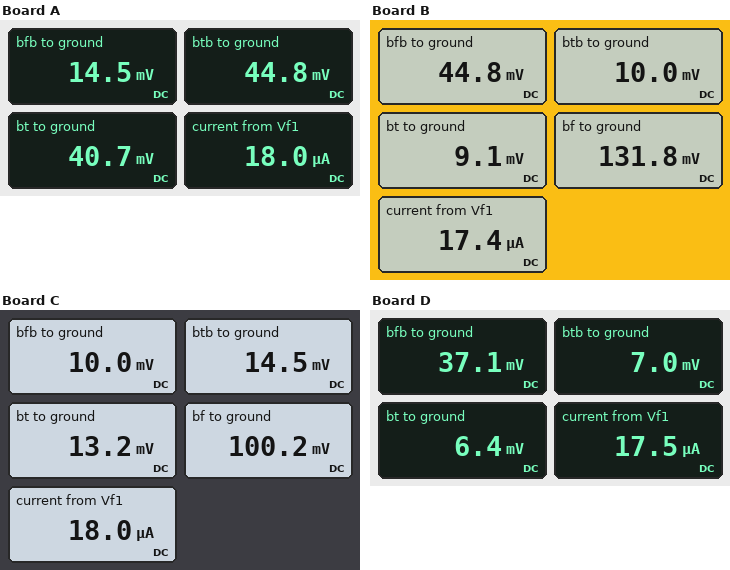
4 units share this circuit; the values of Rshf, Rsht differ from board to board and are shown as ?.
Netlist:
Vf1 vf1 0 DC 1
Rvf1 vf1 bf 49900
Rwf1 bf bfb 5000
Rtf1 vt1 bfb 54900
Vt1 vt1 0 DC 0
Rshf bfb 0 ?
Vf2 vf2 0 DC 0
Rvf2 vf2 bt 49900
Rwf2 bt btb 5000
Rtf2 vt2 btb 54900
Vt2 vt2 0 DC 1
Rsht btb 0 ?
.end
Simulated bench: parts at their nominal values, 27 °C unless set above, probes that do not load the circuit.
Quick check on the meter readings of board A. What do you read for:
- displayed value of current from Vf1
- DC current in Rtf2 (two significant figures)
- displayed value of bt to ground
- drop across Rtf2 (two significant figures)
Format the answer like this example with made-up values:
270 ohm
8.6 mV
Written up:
18.0 µA
17 µA
40.7 mV
960 mV
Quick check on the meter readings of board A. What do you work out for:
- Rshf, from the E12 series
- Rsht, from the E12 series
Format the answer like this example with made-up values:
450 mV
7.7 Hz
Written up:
820 Ω
2.7 kΩ
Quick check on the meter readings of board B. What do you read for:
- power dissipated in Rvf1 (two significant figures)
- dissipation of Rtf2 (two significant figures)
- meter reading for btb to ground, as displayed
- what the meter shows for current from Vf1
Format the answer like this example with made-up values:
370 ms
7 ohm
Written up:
15 µW
18 µW
10.0 mV
17.4 µA
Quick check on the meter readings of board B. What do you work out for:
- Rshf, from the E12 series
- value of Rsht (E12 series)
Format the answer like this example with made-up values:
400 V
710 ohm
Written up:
2.7 kΩ
560 Ω
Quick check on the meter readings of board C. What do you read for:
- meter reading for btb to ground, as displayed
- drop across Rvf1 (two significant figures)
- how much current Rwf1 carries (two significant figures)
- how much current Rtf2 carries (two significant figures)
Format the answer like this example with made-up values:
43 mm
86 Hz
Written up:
14.5 mV
900 mV
18 µA
18 µA
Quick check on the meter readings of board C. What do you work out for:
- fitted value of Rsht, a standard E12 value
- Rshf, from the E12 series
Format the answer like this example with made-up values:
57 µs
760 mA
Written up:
820 Ω
560 Ω
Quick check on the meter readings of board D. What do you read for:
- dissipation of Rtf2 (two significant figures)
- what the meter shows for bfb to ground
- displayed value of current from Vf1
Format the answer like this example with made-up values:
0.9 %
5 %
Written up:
18 µW
37.1 mV
17.5 µA
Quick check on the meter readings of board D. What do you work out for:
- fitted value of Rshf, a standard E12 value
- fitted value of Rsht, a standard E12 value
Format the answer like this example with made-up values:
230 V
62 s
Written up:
2.2 kΩ
390 Ω
